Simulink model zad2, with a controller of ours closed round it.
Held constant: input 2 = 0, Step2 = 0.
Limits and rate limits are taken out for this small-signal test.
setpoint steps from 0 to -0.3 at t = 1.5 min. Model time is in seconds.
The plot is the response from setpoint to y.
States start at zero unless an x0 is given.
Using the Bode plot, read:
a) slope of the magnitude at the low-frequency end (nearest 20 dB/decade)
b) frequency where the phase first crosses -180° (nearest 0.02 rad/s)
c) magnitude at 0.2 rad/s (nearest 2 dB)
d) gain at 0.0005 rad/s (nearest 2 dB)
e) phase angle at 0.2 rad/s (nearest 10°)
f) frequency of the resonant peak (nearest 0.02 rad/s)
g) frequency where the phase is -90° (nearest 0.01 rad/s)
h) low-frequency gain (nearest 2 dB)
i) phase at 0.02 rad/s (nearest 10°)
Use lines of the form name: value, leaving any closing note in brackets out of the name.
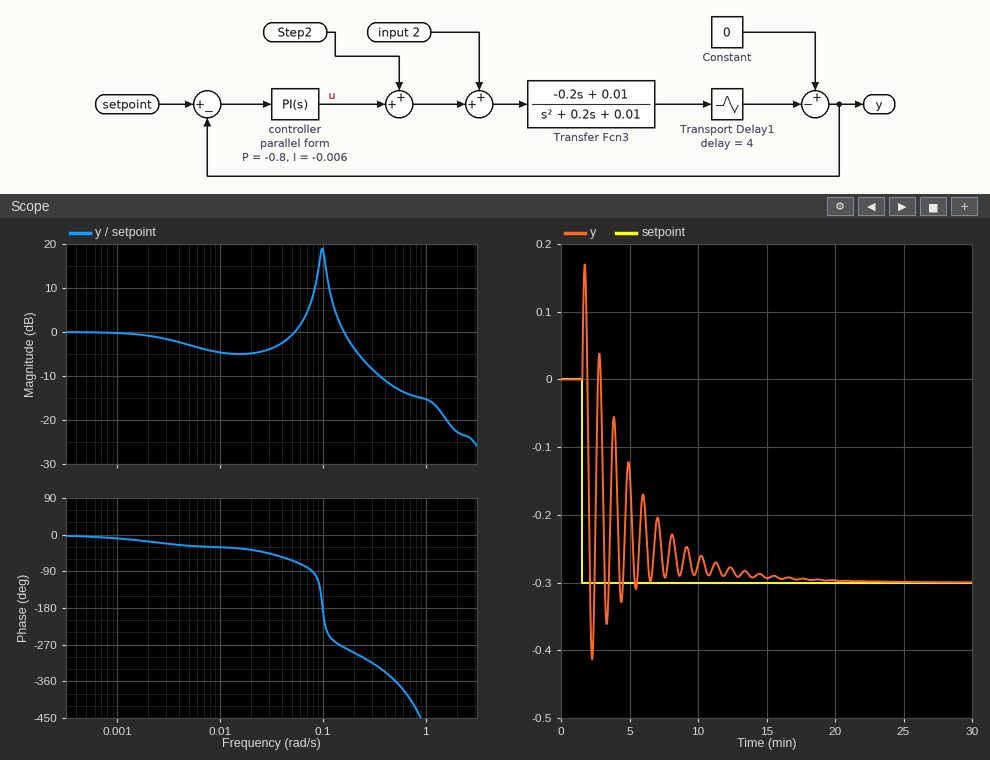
slope of the magnitude at the low-frequency end: 0 dB/decade
frequency where the phase first crosses -180°: 0.10 rad/s
magnitude at 0.2 rad/s: -4 dB
gain at 0.0005 rad/s: 0 dB
phase angle at 0.2 rad/s: -290°
frequency of the resonant peak: 0.10 rad/s
frequency where the phase is -90°: 0.08 rad/s
low-frequency gain: 0 dB
phase at 0.02 rad/s: -40°
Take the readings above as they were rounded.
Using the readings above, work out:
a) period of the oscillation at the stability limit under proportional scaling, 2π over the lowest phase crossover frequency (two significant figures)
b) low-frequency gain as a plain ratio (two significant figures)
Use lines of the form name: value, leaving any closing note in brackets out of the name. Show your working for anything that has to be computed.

period of the oscillation at the stability limit under proportional scaling, 2π over the lowest phase crossover frequency: 2π / 0.1 = 63 s
low-frequency gain as a plain ratio: 10^(0 / 20) = 1.0
